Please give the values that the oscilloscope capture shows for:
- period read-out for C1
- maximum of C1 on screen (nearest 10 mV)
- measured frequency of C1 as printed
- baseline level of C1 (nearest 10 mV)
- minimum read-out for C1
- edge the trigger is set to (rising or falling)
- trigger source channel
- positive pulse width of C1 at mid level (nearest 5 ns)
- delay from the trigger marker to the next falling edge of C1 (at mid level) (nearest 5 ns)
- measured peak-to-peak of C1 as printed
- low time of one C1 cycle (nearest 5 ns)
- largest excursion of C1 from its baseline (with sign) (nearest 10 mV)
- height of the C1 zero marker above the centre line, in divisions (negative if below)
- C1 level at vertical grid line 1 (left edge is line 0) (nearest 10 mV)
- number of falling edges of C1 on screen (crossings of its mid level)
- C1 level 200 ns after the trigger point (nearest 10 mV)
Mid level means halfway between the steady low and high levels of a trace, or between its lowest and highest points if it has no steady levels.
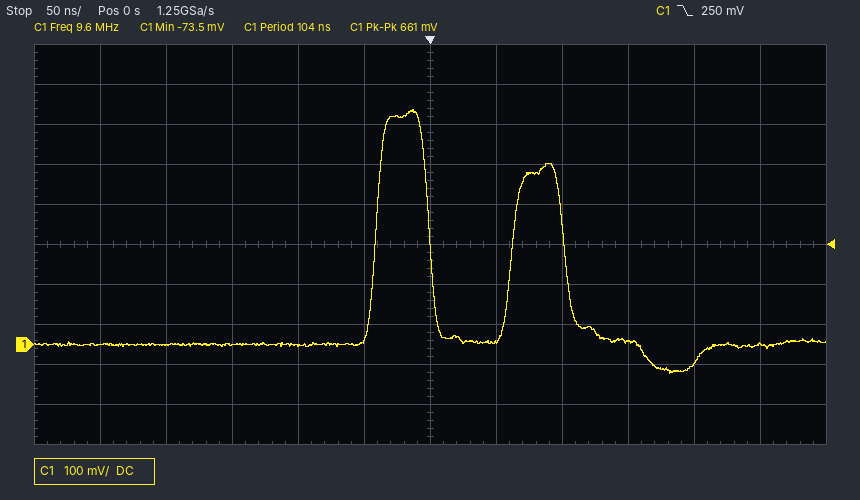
104 ns
590 mV
9.6 MHz
0 mV
-73.5 mV
falling
C1
40 ns
100 ns
661 mV
65 ns
+590 mV
-2.5 div
0 mV
2
-50 mV
